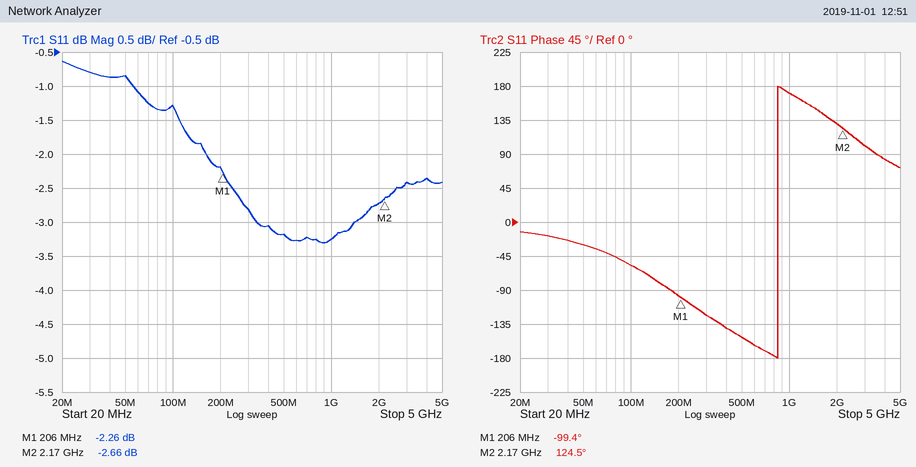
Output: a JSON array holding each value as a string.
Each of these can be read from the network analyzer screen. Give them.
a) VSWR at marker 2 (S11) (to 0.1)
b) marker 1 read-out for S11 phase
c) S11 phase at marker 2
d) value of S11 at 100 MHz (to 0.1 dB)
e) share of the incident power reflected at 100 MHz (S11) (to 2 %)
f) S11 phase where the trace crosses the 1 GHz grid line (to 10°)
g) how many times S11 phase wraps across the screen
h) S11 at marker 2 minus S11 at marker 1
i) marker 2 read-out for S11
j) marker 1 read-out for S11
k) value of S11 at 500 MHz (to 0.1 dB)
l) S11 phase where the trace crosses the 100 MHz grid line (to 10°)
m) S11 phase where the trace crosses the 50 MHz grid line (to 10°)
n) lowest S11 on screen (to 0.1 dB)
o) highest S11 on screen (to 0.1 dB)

["6.6", "-99.4°", "124.5°", "-1.3 dB", "74 %", "170°", "1", "-0.40 dB", "-2.66 dB", "-2.26 dB", "-3.2 dB", "-60°", "-30°", "-3.3 dB", "-0.6 dB"]
